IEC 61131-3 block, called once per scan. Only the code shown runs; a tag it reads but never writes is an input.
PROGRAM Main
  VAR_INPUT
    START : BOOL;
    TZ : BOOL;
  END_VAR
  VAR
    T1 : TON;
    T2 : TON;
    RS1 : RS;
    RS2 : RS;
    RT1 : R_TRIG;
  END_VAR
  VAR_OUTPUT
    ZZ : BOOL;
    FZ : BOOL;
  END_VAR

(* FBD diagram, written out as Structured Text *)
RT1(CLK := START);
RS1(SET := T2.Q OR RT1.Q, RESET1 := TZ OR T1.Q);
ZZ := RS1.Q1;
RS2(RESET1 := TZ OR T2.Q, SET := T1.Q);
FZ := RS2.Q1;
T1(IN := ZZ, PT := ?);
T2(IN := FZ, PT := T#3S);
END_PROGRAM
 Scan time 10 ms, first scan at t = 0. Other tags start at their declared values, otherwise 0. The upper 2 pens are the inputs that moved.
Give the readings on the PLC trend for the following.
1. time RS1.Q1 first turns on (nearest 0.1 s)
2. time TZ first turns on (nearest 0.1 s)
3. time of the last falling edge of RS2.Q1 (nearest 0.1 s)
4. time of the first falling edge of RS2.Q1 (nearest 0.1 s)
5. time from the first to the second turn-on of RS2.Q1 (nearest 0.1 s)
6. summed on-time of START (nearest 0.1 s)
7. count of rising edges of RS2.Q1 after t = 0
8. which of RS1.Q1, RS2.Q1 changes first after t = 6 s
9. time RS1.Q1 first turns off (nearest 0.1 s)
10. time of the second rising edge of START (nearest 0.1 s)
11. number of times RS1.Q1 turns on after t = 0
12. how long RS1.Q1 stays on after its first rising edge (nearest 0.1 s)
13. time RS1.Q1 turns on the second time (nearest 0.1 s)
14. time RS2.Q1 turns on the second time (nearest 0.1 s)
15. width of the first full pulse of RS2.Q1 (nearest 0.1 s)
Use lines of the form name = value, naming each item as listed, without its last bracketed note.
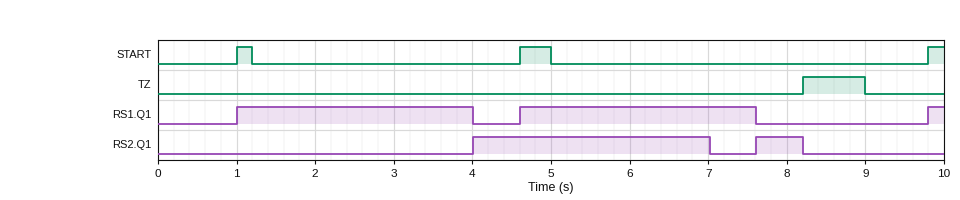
time RS1.Q1 first turns on = 1.0 s
time TZ first turns on = 8.2 s
time of the last falling edge of RS2.Q1 = 8.2 s
time of the first falling edge of RS2.Q1 = 7.0 s
time from the first to the second turn-on of RS2.Q1 = 3.6 s
summed on-time of START = 0.8 s
count of rising edges of RS2.Q1 after t = 0 = 2
which of RS1.Q1, RS2.Q1 changes first after t = 6 s = RS2.Q1
time RS1.Q1 first turns off = 4.0 s
time of the second rising edge of START = 4.6 s
number of times RS1.Q1 turns on after t = 0 = 3
how long RS1.Q1 stays on after its first rising edge = 3.0 s
time RS1.Q1 turns on the second time = 4.6 s
time RS2.Q1 turns on the second time = 7.6 s
width of the first full pulse of RS2.Q1 = 3.0 s
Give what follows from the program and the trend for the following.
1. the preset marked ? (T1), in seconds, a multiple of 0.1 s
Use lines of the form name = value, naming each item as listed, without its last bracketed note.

the preset marked ? (T1), in seconds, a multiple of 0.1 s = 3.0 s
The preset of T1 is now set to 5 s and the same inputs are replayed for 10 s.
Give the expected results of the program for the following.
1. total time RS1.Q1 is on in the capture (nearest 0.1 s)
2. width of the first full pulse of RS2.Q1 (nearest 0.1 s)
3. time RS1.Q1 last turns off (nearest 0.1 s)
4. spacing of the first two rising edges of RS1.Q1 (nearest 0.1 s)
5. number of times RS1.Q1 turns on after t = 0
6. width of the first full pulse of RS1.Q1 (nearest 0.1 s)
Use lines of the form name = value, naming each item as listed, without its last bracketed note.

total time RS1.Q1 is on in the capture = 5.2 s
width of the first full pulse of RS2.Q1 = 2.2 s
time RS1.Q1 last turns off = 6.0 s
spacing of the first two rising edges of RS1.Q1 = 8.8 s
number of times RS1.Q1 turns on after t = 0 = 2
width of the first full pulse of RS1.Q1 = 5.0 s
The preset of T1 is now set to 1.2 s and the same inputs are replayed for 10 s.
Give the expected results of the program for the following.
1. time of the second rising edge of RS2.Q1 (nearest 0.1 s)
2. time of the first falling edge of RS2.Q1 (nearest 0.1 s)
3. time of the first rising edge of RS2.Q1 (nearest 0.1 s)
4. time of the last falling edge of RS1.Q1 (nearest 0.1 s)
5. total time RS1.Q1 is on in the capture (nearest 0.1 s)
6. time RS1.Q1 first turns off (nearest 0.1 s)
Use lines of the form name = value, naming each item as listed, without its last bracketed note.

time of the second rising edge of RS2.Q1 = 5.8 s
time of the first falling edge of RS2.Q1 = 5.2 s
time of the first rising edge of RS2.Q1 = 2.2 s
time of the last falling edge of RS1.Q1 = 5.8 s
total time RS1.Q1 is on in the capture = 2.6 s
time RS1.Q1 first turns off = 2.2 s
